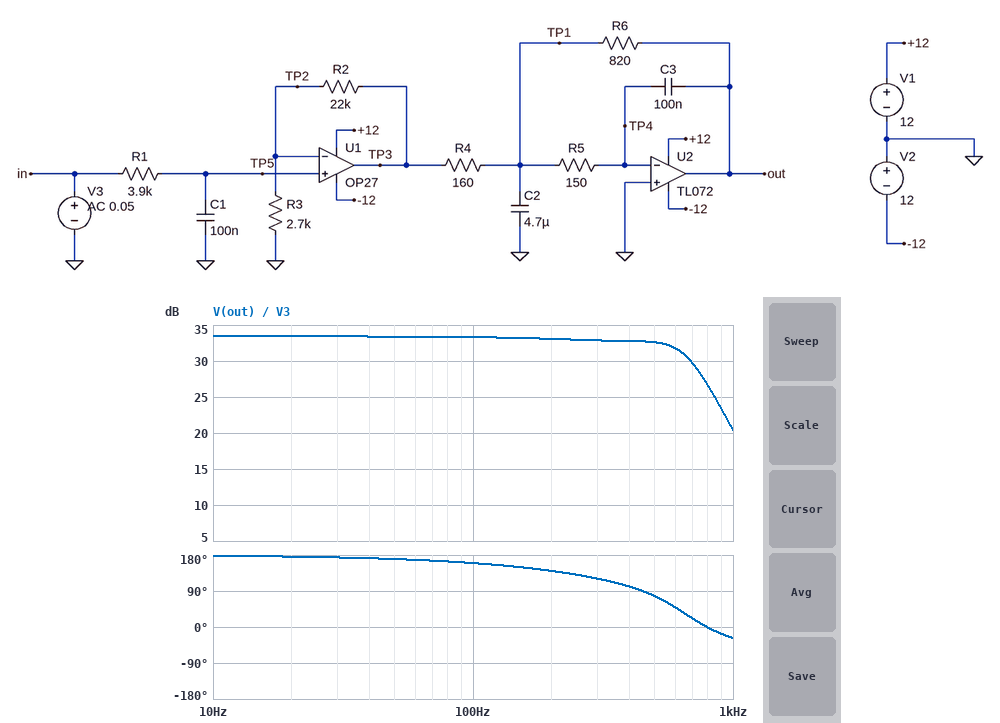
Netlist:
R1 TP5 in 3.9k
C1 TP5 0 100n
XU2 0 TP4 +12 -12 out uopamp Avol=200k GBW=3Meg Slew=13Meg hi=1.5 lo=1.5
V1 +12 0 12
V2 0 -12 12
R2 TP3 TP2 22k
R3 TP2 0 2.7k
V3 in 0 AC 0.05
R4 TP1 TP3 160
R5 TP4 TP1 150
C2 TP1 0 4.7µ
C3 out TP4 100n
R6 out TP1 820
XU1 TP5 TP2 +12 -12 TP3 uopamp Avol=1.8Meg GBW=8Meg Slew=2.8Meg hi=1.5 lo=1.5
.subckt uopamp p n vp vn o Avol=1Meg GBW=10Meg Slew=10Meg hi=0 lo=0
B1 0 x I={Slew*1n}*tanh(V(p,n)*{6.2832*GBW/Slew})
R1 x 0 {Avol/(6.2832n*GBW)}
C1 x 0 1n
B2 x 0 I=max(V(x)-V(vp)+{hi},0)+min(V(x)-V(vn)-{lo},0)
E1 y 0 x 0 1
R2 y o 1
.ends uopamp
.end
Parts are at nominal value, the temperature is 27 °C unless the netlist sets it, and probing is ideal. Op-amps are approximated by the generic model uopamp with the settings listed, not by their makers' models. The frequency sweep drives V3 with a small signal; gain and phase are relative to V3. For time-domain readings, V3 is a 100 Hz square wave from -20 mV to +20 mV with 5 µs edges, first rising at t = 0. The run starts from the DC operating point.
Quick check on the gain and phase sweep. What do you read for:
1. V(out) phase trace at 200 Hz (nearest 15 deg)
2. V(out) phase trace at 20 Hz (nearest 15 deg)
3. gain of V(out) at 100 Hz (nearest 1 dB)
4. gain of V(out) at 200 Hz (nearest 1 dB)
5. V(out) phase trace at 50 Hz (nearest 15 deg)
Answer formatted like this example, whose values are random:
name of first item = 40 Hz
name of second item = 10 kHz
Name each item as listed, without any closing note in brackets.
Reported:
V(out) phase trace at 200 Hz = 135 deg
V(out) phase trace at 20 Hz = 180 deg
gain of V(out) at 100 Hz = 33 dB
gain of V(out) at 200 Hz = 33 dB
V(out) phase trace at 50 Hz = 165 deg
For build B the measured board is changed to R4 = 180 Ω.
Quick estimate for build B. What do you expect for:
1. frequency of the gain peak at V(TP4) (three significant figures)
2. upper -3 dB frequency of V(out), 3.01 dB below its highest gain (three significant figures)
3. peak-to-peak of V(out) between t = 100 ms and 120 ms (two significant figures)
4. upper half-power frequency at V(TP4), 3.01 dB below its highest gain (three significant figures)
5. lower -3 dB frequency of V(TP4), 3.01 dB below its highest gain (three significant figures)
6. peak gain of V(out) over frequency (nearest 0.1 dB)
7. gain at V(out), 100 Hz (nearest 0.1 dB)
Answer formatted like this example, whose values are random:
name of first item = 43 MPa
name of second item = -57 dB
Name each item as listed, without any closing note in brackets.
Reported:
frequency of the gain peak at V(TP4) = 606 Hz
upper -3 dB frequency of V(out), 3.01 dB below its highest gain = 688 Hz
peak-to-peak of V(out) between t = 100 ms and 120 ms = 1.9 V
upper half-power frequency at V(TP4), 3.01 dB below its highest gain = 813 Hz
lower -3 dB frequency of V(TP4), 3.01 dB below its highest gain = 391 Hz
peak gain of V(out) over frequency = 32.4 dB
gain at V(out), 100 Hz = 32.3 dB
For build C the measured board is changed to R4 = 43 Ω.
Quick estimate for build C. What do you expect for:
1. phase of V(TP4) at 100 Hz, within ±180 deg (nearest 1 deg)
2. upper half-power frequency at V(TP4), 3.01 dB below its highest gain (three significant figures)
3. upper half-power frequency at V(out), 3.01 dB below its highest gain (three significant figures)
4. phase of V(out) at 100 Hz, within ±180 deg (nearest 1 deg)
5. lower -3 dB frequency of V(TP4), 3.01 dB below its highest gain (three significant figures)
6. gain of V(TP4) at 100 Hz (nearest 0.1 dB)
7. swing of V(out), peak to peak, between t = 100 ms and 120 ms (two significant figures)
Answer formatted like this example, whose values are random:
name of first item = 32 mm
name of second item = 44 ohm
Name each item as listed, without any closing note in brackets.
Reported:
phase of V(TP4) at 100 Hz, within ±180 deg = 54 deg
upper half-power frequency at V(TP4), 3.01 dB below its highest gain = 826 Hz
upper half-power frequency at V(out), 3.01 dB below its highest gain = 333 Hz
phase of V(out) at 100 Hz, within ±180 deg = 152 deg
lower -3 dB frequency of V(TP4), 3.01 dB below its highest gain = 202 Hz
gain of V(TP4) at 100 Hz = -44.9 dB
swing of V(out), peak to peak, between t = 100 ms and 120 ms = 7.0 V
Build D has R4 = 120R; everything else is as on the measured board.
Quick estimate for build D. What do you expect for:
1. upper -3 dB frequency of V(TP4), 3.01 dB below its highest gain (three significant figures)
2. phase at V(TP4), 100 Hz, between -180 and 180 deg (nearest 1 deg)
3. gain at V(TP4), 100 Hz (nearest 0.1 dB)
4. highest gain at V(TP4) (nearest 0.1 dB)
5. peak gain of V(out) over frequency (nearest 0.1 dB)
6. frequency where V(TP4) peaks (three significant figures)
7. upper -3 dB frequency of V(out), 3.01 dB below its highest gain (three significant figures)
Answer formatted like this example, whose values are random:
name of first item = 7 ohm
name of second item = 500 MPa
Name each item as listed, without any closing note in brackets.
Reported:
upper -3 dB frequency of V(TP4), 3.01 dB below its highest gain = 827 Hz
phase at V(TP4), 100 Hz, between -180 and 180 deg = 60 deg
gain at V(TP4), 100 Hz = -53.6 dB
highest gain at V(TP4) = -40.8 dB
peak gain of V(out) over frequency = 35.9 dB
frequency where V(TP4) peaks = 583 Hz
upper -3 dB frequency of V(out), 3.01 dB below its highest gain = 614 Hz
